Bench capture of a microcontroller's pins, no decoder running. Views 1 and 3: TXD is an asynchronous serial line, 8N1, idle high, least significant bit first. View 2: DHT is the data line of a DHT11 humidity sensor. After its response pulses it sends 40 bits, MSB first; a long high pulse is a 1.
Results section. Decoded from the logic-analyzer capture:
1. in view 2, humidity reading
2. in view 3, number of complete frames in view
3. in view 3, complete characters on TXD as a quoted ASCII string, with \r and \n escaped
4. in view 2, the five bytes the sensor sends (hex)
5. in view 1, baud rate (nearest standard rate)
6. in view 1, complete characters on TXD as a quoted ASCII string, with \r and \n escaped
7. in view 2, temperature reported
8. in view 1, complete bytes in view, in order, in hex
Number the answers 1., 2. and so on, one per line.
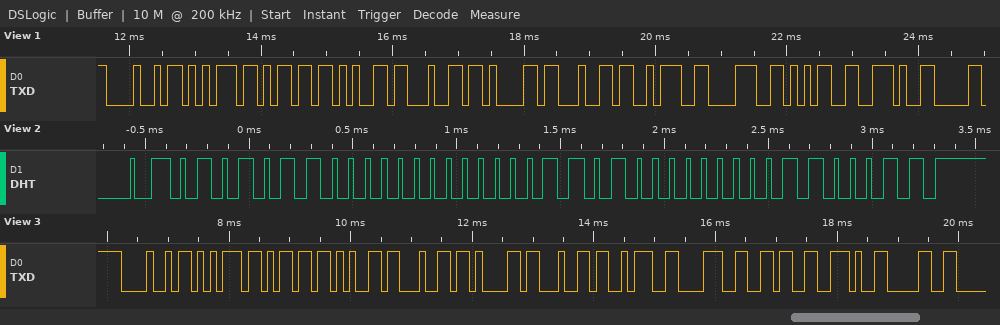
1. 86 %
2. 12
3. "Humedad:86.0"
4. 56 00 0D 00 63
5. 9600 baud
6. "Humedad:85."
7. 13.0 °C
8. 48 75 6D 65 64 61 64 3A 38 35 2E
